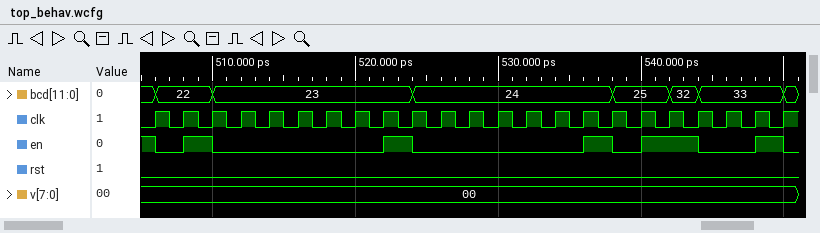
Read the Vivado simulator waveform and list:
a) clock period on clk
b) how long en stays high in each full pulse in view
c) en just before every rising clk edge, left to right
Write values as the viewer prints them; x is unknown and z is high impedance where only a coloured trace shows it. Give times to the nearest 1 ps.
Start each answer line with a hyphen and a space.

- 2 ps
- 2 ps, 2 ps, 2 ps, 4 ps, 2 ps
- 1 0 1 0 0 0 0 0 0 1 0 0 0 0 0 0 1 0 1 1 0 0 1
